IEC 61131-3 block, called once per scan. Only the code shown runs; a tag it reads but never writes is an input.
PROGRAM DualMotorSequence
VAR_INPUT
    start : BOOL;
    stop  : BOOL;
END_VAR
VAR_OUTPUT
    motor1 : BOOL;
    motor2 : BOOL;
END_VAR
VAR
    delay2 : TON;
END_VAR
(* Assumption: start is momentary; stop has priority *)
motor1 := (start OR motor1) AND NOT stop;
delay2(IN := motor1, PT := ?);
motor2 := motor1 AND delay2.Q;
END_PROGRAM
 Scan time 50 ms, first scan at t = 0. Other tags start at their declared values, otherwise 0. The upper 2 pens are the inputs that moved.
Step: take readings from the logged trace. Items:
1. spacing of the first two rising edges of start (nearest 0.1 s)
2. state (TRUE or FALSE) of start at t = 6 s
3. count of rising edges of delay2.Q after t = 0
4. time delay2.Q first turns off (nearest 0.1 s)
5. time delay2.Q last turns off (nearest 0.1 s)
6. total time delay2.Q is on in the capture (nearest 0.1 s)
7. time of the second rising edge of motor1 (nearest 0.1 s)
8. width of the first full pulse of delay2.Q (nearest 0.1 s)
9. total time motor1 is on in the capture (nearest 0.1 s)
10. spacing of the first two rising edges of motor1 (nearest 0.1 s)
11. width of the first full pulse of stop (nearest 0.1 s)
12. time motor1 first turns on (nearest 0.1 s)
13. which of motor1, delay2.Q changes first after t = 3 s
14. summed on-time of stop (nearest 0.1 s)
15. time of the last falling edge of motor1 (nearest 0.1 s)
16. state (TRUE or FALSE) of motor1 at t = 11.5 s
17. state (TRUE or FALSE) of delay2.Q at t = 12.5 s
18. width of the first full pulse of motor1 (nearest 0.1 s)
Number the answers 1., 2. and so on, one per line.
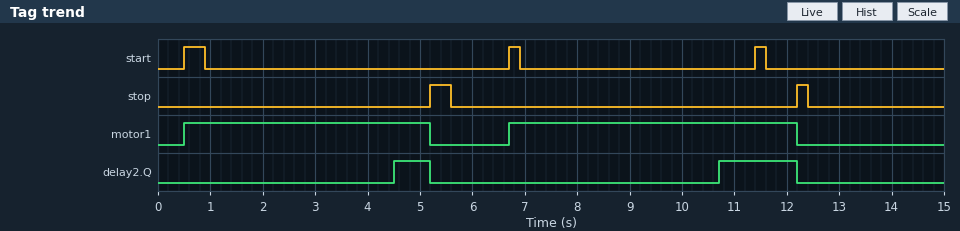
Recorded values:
1. 6.2 s
2. FALSE
3. 2
4. 5.2 s
5. 12.2 s
6. 2.2 s
7. 6.7 s
8. 0.7 s
9. 10.2 s
10. 6.2 s
11. 0.4 s
12. 0.5 s
13. delay2.Q
14. 0.6 s
15. 12.2 s
16. TRUE
17. FALSE
18. 4.7 s
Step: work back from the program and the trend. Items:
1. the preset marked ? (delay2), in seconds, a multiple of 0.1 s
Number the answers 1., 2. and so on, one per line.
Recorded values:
1. 4.0 s
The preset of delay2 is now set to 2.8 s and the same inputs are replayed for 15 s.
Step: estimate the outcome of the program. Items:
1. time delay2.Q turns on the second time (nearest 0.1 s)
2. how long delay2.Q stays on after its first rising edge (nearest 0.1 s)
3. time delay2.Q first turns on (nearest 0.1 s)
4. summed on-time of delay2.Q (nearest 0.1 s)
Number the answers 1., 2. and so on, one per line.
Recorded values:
1. 9.5 s
2. 1.9 s
3. 3.3 s
4. 4.6 s
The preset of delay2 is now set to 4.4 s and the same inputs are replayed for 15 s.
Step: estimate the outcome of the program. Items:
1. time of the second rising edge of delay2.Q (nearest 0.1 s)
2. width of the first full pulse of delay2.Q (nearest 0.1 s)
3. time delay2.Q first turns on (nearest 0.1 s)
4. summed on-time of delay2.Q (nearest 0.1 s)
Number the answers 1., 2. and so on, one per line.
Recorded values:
1. 11.1 s
2. 0.3 s
3. 4.9 s
4. 1.4 s
